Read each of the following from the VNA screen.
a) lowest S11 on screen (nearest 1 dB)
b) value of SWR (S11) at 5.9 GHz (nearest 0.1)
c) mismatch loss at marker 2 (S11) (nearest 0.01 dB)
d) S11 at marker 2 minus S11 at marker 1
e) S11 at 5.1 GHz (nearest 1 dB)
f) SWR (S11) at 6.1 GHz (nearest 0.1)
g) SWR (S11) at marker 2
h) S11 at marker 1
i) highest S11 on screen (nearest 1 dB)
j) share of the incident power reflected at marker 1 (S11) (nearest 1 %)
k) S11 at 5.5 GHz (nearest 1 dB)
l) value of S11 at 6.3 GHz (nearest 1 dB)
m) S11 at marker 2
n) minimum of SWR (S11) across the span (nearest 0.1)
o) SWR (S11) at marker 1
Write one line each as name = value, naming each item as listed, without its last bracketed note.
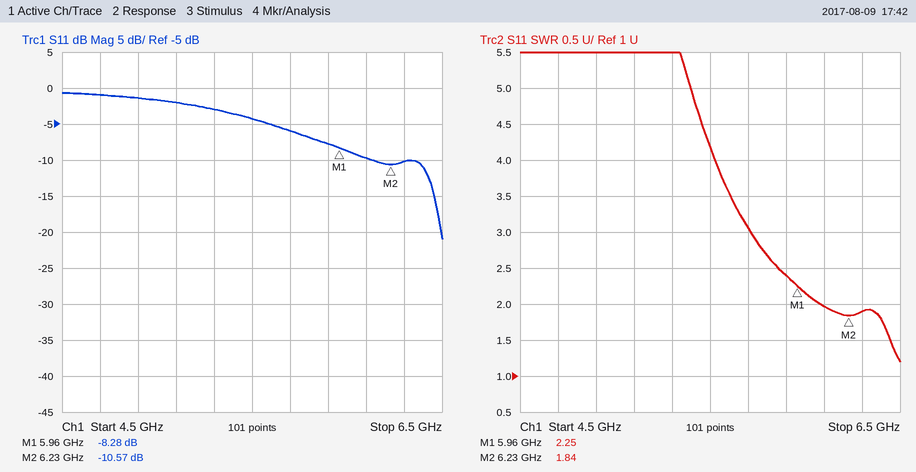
lowest S11 on screen = -21 dB
value of SWR (S11) at 5.9 GHz = 2.4
mismatch loss at marker 2 (S11) = 0.40 dB
S11 at marker 2 minus S11 at marker 1 = -2.29 dB
S11 at 5.1 GHz = -2 dB
SWR (S11) at 6.1 GHz = 2.0
SWR (S11) at marker 2 = 1.84
S11 at marker 1 = -8.28 dB
highest S11 on screen = -1 dB
share of the incident power reflected at marker 1 (S11) = 15 %
S11 at 5.5 GHz = -4 dB
value of S11 at 6.3 GHz = -10 dB
S11 at marker 2 = -10.57 dB
minimum of SWR (S11) across the span = 1.2
SWR (S11) at marker 1 = 2.25
